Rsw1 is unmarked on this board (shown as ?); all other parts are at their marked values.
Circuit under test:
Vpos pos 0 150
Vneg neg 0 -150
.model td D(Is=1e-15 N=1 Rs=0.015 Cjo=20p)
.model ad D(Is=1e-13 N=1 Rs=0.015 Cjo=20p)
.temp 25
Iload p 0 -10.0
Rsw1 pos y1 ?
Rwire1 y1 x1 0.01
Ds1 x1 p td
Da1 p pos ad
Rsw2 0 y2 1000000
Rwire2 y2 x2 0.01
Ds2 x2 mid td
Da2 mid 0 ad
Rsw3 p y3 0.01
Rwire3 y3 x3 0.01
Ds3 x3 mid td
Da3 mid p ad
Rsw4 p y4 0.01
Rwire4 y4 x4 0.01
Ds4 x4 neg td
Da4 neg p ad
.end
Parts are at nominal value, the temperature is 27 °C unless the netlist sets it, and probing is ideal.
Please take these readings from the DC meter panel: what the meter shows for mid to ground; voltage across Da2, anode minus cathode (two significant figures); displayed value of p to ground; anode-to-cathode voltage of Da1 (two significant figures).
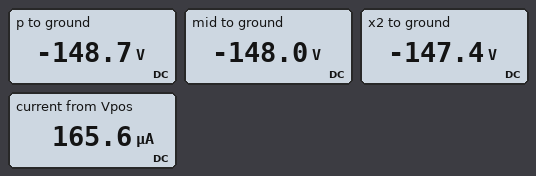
-148.0 V
-150 V
-148.7 V
-300 V
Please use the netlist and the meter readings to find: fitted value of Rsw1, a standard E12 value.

1.8 MΩ
